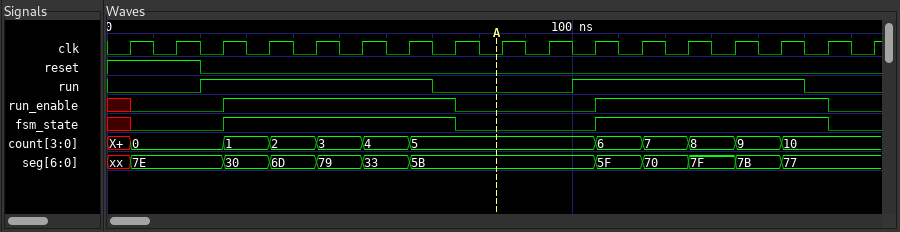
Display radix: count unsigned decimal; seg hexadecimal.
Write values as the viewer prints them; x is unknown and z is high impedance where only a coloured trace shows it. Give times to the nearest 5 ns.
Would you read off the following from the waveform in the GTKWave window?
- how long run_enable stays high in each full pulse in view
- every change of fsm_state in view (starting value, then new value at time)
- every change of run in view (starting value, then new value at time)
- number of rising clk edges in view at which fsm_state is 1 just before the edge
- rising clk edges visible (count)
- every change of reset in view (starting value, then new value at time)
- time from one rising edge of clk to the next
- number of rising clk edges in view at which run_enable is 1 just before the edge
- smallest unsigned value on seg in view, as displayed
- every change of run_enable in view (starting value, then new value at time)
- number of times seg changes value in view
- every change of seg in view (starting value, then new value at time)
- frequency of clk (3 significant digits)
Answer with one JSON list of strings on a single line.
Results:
["50 ns, 50 ns", "x, 0 at 5 ns, 1 at 25 ns, 0 at 75 ns, 1 at 105 ns, 0 at 155 ns", "0, 1 at 20 ns, 0 at 70 ns, 1 at 100 ns, 0 at 150 ns", "10", "17", "1, 0 at 20 ns", "10 ns", "10", "30", "x, 0 at 5 ns, 1 at 25 ns, 0 at 75 ns, 1 at 105 ns, 0 at 155 ns", "11", "xx, 7E at 5 ns, 30 at 25 ns, 6D at 35 ns, 79 at 45 ns, 33 at 55 ns, 5B at 65 ns, 5F at 105 ns, 70 at 115 ns, 7F at 125 ns, 7B at 135 ns, 77 at 145 ns", "100 MHz"]
